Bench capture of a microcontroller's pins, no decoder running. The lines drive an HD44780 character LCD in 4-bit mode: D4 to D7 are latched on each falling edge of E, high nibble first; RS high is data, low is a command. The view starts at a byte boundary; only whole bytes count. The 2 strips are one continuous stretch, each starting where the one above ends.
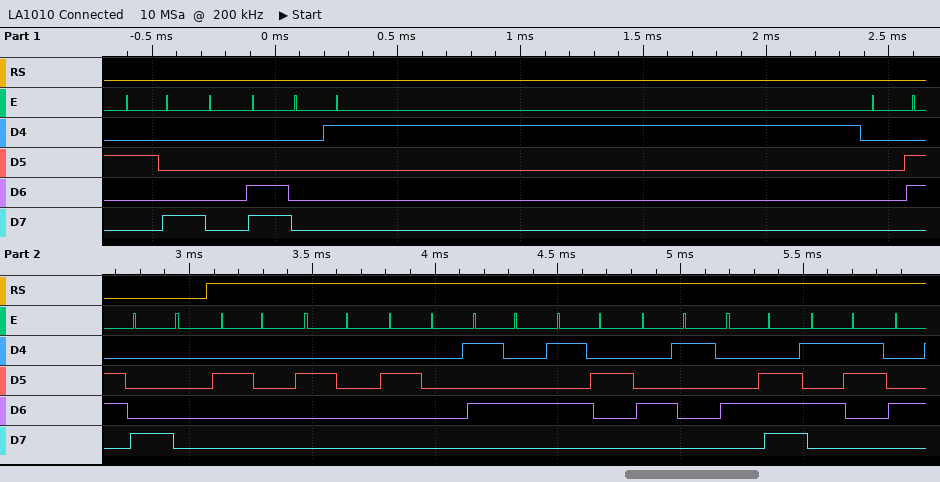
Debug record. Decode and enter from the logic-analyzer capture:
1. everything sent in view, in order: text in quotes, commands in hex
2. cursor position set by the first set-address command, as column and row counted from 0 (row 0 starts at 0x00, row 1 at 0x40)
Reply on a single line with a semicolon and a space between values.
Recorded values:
0x28 0x0C 0x01 0x06 0x80 "   TRANS"; column 0, row 0
